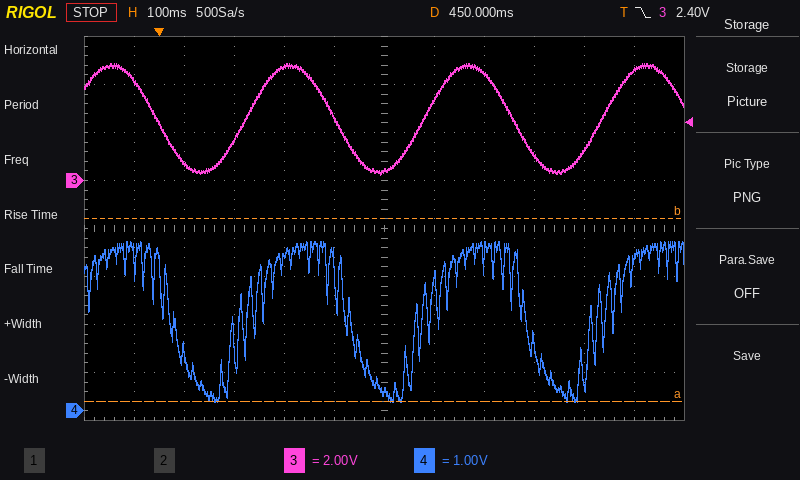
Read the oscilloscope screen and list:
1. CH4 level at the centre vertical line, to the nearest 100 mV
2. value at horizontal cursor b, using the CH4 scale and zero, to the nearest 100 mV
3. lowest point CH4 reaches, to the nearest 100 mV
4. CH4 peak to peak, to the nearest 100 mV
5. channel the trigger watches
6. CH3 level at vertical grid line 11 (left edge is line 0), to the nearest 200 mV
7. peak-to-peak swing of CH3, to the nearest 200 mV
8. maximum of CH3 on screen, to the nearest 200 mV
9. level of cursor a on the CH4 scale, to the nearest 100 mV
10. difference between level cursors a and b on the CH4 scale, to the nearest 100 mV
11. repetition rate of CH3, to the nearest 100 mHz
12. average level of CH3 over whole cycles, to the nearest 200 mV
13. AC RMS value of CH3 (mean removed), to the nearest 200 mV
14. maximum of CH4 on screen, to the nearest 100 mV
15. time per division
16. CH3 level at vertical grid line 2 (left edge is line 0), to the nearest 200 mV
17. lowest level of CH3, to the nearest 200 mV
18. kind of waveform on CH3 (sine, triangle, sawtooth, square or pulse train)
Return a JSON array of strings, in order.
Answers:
["400 mV", "4.0 V", "200 mV", "3.3 V", "CH3", "4.6 V", "4.6 V", "4.8 V", "200 mV", "3.8 V", "2.8 Hz", "2.6 V", "1.6 V", "3.5 V", "100 ms", "800 mV", "200 mV", "sine"]
